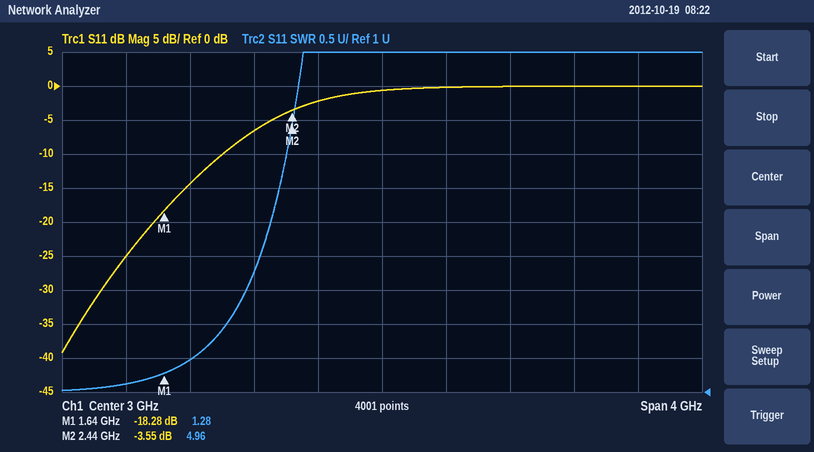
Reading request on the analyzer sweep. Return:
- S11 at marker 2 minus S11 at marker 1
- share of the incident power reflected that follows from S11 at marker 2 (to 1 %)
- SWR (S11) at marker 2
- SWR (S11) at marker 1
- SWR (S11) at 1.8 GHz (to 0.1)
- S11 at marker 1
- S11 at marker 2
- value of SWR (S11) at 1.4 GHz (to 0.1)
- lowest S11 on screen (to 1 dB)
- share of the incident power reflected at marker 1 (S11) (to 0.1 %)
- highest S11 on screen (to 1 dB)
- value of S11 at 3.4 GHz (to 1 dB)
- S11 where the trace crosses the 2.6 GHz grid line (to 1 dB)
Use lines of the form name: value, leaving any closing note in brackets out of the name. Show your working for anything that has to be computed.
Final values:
S11 at marker 2 minus S11 at marker 1: -3.55 − (-18.28) = 14.73 dB
share of the incident power reflected that follows from S11 at marker 2: 10^(-3.55/10) ≈ 44 %
SWR (S11) at marker 2: 4.96
SWR (S11) at marker 1: 1.28
SWR (S11) at 1.8 GHz: 1.5
S11 at marker 1: -18.28 dB
S11 at marker 2: -3.55 dB
value of SWR (S11) at 1.4 GHz: 1.1
lowest S11 on screen: -39 dB
share of the incident power reflected at marker 1 (S11): 10^(-18.28/10) ≈ 1.5 %
highest S11 on screen: 0 dB
value of S11 at 3.4 GHz: 0 dB
S11 where the trace crosses the 2.6 GHz grid line: -2 dB
